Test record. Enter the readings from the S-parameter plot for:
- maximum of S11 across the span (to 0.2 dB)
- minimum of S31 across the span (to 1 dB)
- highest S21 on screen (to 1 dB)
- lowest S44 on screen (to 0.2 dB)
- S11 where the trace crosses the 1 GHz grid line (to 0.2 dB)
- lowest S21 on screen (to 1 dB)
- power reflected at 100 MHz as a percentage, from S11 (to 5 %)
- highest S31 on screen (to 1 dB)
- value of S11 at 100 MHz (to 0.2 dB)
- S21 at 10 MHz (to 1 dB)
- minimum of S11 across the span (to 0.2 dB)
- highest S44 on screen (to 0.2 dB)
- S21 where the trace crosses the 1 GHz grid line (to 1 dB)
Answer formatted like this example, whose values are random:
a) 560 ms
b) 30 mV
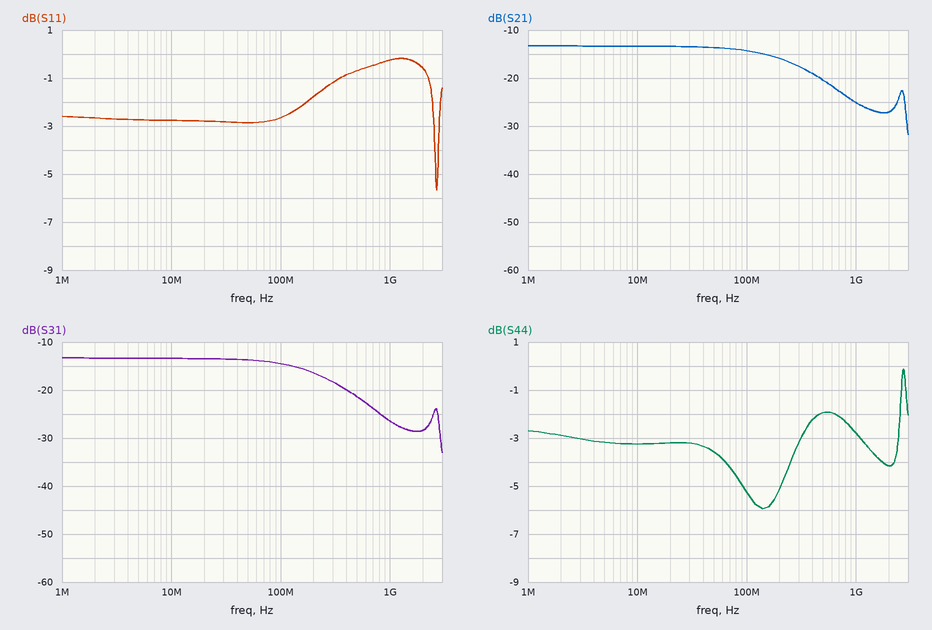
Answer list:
a) -0.2 dB
b) -33 dB
c) -13 dB
d) -6.0 dB
e) -0.2 dB
f) -32 dB
g) 55 %
h) -13 dB
i) -2.6 dB
j) -13 dB
k) -5.6 dB
l) -0.2 dB
m) -25 dB
